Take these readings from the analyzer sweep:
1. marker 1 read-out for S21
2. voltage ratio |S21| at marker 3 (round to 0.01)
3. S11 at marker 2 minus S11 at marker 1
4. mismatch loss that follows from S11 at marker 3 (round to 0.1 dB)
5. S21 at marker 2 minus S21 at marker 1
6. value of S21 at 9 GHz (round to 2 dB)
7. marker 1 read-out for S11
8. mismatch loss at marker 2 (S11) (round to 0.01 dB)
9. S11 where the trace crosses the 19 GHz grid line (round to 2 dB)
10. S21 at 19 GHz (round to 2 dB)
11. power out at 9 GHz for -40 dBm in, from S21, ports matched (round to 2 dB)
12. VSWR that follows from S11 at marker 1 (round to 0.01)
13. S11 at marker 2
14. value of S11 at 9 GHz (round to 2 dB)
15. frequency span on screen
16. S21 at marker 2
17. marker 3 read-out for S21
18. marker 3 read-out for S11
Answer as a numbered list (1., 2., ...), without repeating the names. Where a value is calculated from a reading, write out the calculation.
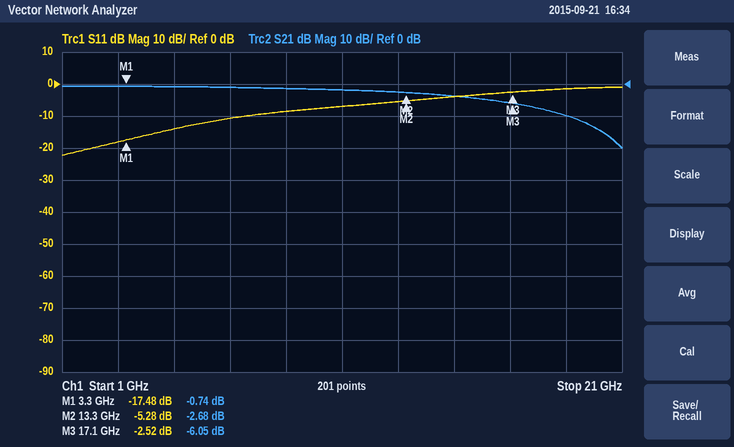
1. -0.74 dB
2. 10^(-6.05/20) ≈ 0.50
3. -5.28 − (-17.48) = 12.20 dB
4. −10 log10(1 − 10^(-2.52/10)) ≈ 3.6 dB
5. -2.68 − (-0.74) = -1.94 dB
6. -2 dB
7. -17.48 dB
8. −10 log10(1 − 10^(-5.28/10)) ≈ 1.53 dB
9. -2 dB
10. -10 dB
11. -40 dBm + (-2 dB) = -42 dBm
12. (1 + 0.1337)/(1 − 0.1337) ≈ 1.31
13. -5.28 dB
14. -8 dB
15. 20 GHz
16. -2.68 dB
17. -6.05 dB
18. -2.52 dB
